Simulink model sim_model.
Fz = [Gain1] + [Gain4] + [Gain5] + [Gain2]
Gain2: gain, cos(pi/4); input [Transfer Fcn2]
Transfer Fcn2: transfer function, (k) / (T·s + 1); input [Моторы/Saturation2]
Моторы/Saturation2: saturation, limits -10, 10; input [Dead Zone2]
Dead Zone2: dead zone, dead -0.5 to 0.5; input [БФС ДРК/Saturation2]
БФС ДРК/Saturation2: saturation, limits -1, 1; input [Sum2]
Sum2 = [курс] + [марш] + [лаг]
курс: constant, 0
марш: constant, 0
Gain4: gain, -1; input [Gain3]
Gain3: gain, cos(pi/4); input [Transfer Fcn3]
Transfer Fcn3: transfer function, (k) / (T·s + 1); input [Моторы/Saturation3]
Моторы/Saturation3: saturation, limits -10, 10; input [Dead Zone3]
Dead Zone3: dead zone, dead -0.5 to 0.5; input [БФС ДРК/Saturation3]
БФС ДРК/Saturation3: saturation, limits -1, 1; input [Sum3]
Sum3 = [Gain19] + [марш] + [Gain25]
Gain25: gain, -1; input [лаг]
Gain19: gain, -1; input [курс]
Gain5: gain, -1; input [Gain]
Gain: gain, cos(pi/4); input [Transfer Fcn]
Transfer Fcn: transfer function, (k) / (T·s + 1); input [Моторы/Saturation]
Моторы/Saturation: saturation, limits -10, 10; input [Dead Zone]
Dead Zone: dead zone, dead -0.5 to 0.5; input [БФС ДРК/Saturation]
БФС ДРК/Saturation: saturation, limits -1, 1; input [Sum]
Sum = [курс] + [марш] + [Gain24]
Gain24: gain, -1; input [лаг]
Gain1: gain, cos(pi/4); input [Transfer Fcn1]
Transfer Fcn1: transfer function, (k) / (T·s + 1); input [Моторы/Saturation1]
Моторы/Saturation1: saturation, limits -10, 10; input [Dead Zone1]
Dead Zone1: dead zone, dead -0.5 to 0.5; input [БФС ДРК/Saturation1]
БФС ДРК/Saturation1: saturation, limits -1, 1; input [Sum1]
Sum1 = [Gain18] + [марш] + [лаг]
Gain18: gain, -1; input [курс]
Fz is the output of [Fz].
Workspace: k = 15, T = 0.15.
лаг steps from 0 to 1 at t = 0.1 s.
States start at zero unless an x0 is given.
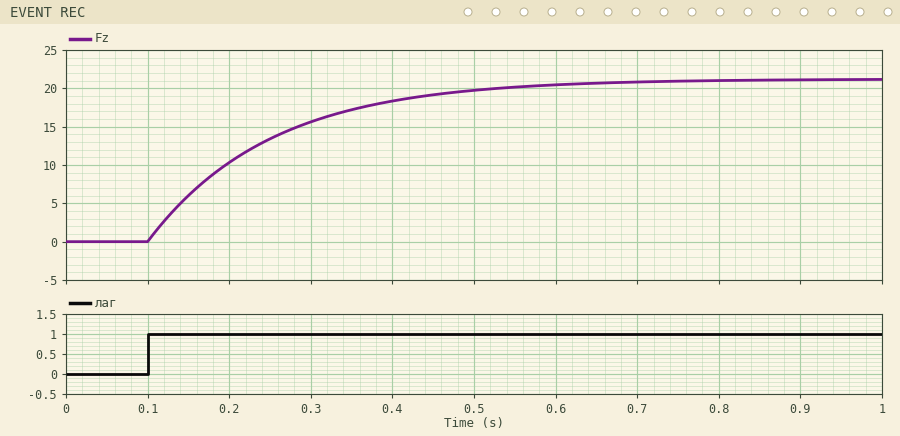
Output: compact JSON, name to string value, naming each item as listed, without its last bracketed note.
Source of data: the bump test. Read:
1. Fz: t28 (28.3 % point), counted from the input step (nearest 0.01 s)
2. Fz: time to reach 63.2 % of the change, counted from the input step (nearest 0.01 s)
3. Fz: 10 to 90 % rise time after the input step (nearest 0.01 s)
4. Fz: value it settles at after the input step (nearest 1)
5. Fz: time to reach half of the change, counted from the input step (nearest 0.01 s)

{"Fz: t28 (28.3 % point), counted from the input step": "0.05 s", "Fz: time to reach 63.2 % of the change, counted from the input step": "0.15 s", "Fz: 10 to 90 % rise time after the input step": "0.33 s", "Fz: value it settles at after the input step": "21", "Fz: time to reach half of the change, counted from the input step": "0.10 s"}
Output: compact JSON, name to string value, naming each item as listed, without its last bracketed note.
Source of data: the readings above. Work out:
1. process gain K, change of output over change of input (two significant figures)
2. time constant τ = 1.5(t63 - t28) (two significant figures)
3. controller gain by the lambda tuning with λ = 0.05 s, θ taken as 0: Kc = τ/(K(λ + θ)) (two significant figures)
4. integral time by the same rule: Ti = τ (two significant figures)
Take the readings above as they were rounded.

{"process gain K, change of output over change of input": "21", "time constant τ = 1.5(t63 - t28)": "0.15 s", "controller gain by the lambda tuning with λ = 0.05 s, θ taken as 0: Kc = τ/(K(λ + θ))": "0.14", "integral time by the same rule: Ti = τ": "0.15 s"}
